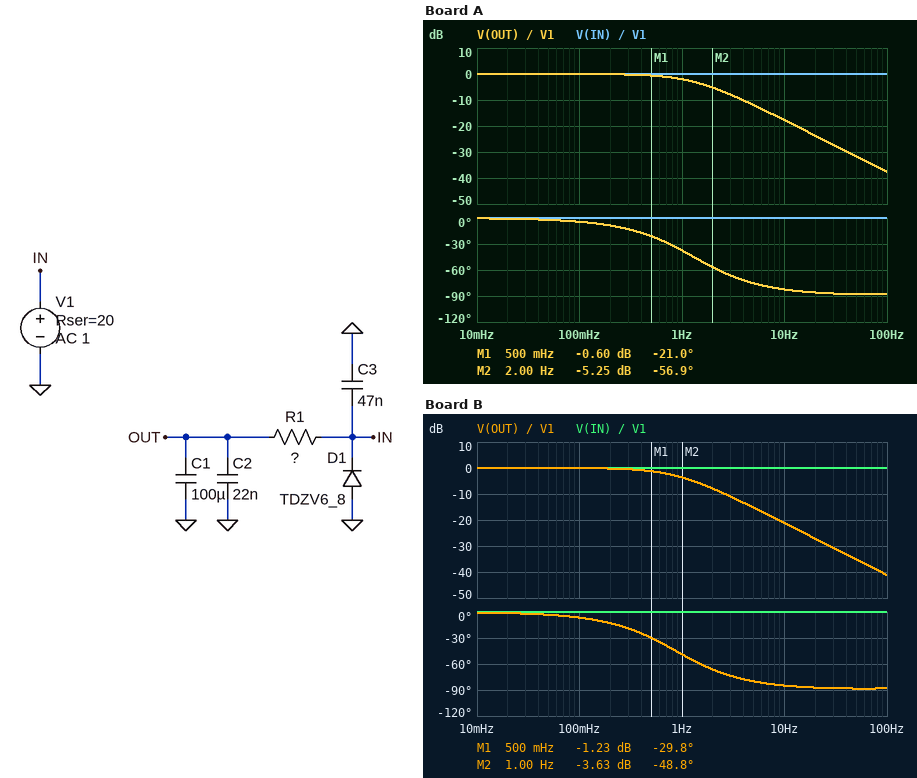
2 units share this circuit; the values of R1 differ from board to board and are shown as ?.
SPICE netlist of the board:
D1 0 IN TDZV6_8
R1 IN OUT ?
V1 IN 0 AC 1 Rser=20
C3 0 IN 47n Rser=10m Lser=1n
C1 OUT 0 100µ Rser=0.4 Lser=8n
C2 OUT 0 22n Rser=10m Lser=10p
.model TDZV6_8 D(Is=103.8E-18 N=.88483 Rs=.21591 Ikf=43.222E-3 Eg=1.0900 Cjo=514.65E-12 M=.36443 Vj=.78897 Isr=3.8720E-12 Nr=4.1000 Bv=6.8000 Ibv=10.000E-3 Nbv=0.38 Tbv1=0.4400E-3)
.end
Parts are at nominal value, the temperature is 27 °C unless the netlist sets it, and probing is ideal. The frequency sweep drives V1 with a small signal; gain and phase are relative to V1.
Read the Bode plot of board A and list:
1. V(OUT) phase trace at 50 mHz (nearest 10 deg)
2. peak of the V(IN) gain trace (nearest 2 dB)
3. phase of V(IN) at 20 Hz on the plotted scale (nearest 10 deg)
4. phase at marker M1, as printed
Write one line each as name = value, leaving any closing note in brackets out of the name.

V(OUT) phase trace at 50 mHz = 0 deg
peak of the V(IN) gain trace = 0 dB
phase of V(IN) at 20 Hz on the plotted scale = 0 deg
phase at marker M1, as printed = -21.0 deg
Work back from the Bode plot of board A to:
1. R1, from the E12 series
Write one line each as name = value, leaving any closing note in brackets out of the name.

R1, from the E12 series = 1.2 kΩ
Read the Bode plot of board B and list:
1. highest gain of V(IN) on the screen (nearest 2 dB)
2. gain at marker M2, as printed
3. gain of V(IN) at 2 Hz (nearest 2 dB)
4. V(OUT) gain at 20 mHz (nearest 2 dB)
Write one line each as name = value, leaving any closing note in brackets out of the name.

highest gain of V(IN) on the screen = 0 dB
gain at marker M2, as printed = -3.63 dB
gain of V(IN) at 2 Hz = 0 dB
V(OUT) gain at 20 mHz = 0 dB
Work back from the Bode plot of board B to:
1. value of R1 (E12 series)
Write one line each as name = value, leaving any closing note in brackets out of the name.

value of R1 = 1.8 kΩ
